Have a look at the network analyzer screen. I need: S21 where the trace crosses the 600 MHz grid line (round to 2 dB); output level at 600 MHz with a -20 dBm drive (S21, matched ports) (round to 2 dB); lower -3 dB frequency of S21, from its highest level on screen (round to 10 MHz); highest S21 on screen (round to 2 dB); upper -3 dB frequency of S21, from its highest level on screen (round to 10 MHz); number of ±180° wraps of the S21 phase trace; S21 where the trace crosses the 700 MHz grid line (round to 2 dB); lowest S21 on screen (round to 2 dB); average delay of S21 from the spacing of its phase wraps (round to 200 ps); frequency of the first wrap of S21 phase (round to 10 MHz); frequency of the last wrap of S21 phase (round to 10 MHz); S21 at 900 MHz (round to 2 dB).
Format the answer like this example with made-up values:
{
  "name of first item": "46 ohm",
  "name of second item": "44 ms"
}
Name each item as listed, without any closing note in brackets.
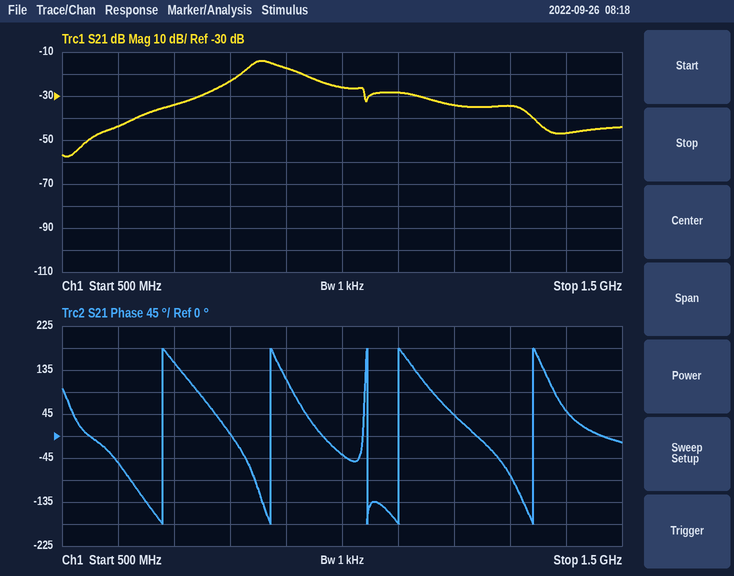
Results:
{
  "S21 where the trace crosses the 600 MHz grid line": "-44 dB",
  "output level at 600 MHz with a -20 dBm drive (S21, matched ports)": "-64 dBm",
  "lower -3 dB frequency of S21, from its highest level on screen": "830 MHz",
  "highest S21 on screen": "-14 dB",
  "upper -3 dB frequency of S21, from its highest level on screen": "900 MHz",
  "number of ±180° wraps of the S21 phase trace": "5",
  "S21 where the trace crosses the 700 MHz grid line": "-34 dB",
  "lowest S21 on screen": "-58 dB",
  "average delay of S21 from the spacing of its phase wraps": "6.0 ns",
  "frequency of the first wrap of S21 phase": "680 MHz",
  "frequency of the last wrap of S21 phase": "1.34 GHz",
  "S21 at 900 MHz": "-18 dB"
}
